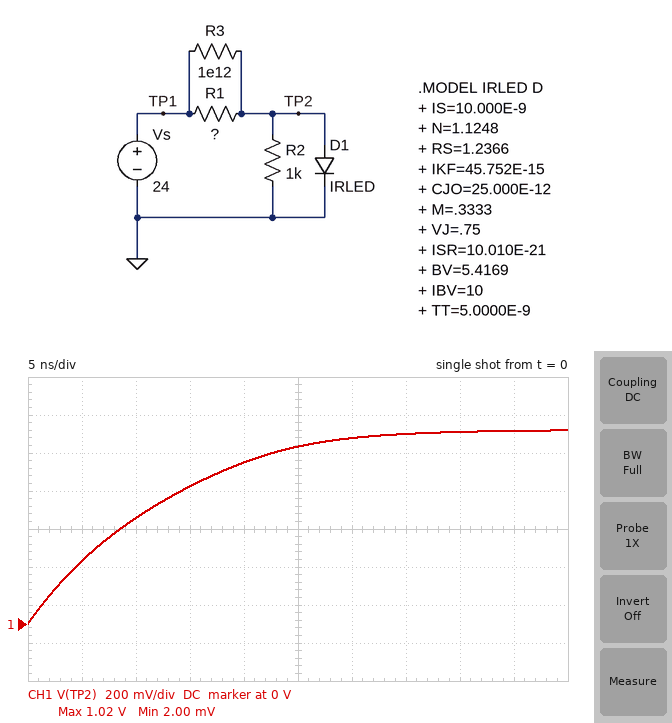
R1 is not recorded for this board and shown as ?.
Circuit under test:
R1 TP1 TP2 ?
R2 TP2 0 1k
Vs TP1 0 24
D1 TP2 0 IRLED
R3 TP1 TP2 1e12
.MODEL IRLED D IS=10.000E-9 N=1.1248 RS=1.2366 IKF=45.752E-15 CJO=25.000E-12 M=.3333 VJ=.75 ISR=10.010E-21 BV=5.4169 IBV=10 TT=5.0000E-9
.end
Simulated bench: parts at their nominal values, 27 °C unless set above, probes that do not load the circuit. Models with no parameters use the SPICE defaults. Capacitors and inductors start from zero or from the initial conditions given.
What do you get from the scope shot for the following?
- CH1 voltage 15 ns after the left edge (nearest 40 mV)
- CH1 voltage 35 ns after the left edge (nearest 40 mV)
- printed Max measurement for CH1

720 mV
1.00 V
1.02 V
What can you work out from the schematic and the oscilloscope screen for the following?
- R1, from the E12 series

12 kΩ
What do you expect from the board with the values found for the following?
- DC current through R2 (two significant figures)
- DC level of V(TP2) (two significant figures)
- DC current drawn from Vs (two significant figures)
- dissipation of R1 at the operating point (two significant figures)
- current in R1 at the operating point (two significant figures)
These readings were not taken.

1.0 mA
1.0 V
1.9 mA
44 mW
1.9 mA
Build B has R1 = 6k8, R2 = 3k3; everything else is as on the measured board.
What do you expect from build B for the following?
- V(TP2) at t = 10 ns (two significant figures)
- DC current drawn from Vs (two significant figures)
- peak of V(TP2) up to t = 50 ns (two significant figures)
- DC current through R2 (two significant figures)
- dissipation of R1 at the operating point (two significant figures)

930 mV
3.4 mA
1.1 V
330 µA
77 mW
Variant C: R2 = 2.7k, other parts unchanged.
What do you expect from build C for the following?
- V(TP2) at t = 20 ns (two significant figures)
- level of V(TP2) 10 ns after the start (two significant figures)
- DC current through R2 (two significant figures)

950 mV
610 mV
390 µA
